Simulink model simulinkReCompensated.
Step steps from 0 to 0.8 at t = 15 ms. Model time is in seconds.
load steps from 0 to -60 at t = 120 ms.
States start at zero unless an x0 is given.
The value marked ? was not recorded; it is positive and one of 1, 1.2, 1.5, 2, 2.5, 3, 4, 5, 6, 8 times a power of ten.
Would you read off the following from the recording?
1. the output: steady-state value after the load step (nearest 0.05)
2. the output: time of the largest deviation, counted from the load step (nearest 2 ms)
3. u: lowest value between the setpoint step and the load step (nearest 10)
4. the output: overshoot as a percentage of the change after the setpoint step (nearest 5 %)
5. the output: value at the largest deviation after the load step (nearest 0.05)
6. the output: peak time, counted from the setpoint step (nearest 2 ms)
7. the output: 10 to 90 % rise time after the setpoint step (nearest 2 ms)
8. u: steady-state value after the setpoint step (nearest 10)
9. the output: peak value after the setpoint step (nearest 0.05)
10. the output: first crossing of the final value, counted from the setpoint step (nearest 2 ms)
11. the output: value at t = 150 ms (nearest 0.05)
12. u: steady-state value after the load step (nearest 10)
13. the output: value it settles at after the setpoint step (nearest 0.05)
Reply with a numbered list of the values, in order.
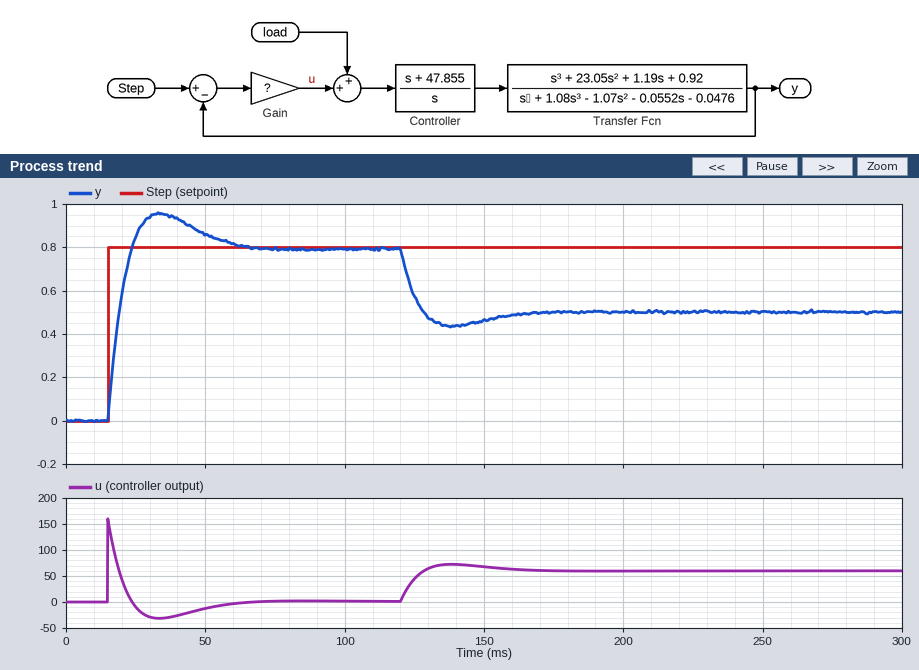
1. 0.50
2. 18 ms
3. -30
4. 20 %
5. 0.45
6. 18 ms
7. 6 ms
8. 0
9. 0.95
10. 8 ms
11. 0.45
12. 60
13. 0.80
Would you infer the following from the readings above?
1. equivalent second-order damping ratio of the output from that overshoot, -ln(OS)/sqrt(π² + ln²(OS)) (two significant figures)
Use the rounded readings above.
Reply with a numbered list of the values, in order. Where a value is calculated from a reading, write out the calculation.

1. ln(0.2) = -1.609; 1.609 / sqrt(9.870 + 2.590) = 0.46
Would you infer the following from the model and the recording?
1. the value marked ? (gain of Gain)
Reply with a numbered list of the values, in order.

1. 200
